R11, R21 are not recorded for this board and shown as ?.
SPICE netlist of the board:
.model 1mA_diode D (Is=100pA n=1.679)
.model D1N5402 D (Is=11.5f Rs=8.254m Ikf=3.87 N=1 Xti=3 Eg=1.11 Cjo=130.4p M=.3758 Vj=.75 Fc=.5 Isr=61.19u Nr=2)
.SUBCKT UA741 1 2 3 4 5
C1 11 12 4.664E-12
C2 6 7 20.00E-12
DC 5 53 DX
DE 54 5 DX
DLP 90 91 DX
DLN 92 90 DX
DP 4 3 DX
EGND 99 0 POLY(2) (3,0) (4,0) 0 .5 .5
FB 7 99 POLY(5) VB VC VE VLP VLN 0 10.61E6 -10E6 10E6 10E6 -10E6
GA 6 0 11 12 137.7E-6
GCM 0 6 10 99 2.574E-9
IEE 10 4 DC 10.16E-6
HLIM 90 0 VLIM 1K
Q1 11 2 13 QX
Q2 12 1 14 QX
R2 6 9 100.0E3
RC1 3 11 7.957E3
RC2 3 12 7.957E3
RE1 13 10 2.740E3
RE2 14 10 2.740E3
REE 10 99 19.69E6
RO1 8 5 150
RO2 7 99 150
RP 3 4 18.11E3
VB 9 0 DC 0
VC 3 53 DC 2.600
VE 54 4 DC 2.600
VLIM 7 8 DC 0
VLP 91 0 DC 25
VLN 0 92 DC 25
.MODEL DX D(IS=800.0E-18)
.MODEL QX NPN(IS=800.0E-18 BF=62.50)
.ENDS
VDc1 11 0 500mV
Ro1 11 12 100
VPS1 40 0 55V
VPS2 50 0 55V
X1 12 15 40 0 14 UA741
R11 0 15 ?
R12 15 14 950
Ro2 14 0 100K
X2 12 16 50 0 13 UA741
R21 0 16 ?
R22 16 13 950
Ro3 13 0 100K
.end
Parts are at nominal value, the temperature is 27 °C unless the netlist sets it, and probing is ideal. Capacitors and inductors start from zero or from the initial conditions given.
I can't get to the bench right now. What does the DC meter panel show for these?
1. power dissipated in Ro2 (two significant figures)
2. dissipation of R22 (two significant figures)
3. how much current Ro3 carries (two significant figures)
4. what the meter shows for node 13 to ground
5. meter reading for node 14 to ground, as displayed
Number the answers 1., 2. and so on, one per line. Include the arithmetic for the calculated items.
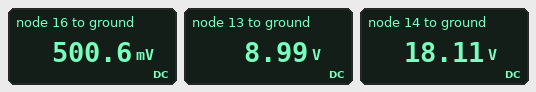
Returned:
1. (18.11 V)^2 / 100 kΩ = 3.3 mW
2. (8.99 V - 500.6 mV)^2 / 950 Ω = 76 mW
3. (8.99 V) / 100 kΩ = 90 µA
4. 8.99 V
5. 18.11 V
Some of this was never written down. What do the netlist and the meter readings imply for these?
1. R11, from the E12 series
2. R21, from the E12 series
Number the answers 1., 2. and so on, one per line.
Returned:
1. 27 Ω
2. 56 Ω
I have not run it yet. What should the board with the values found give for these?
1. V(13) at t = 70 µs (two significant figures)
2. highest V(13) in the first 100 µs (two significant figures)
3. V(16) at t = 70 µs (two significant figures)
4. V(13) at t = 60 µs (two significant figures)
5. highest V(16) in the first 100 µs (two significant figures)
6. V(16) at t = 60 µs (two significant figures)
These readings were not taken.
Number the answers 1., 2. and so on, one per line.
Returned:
1. 9.0 V
2. 9.0 V
3. 500 mV
4. 9.0 V
5. 500 mV
6. 500 mV
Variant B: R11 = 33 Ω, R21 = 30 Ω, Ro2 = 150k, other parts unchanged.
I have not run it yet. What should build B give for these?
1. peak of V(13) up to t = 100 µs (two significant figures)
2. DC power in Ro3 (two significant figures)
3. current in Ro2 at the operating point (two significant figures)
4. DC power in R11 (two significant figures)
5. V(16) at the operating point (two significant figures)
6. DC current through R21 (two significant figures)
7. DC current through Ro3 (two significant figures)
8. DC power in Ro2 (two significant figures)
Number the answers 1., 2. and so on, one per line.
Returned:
1. 16 V
2. 2.7 mW
3. 99 µA
4. 7.6 mW
5. 500 mV
6. 17 mA
7. 160 µA
8. 1.5 mW
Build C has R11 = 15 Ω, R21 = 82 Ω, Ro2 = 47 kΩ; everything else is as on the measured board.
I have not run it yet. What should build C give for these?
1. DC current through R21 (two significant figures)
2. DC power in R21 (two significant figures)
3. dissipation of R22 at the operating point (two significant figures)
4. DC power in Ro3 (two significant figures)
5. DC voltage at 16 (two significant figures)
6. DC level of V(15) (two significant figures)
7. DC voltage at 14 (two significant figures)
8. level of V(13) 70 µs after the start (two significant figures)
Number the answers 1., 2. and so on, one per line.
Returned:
1. 6.1 mA
2. 3.1 mW
3. 35 mW
4. 400 µW
5. 500 mV
6. 380 mV
7. 24 V
8. 6.3 V
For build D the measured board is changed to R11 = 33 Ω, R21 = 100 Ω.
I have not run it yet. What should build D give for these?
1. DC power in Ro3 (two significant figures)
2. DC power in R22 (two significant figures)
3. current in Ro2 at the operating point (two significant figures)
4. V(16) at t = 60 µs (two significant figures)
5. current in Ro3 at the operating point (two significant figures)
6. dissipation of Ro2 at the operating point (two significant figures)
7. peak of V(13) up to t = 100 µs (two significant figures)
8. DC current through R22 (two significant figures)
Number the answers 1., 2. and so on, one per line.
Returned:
1. 280 µW
2. 24 mW
3. 150 µA
4. 500 mV
5. 53 µA
6. 2.2 mW
7. 5.3 V
8. 5.0 mA
